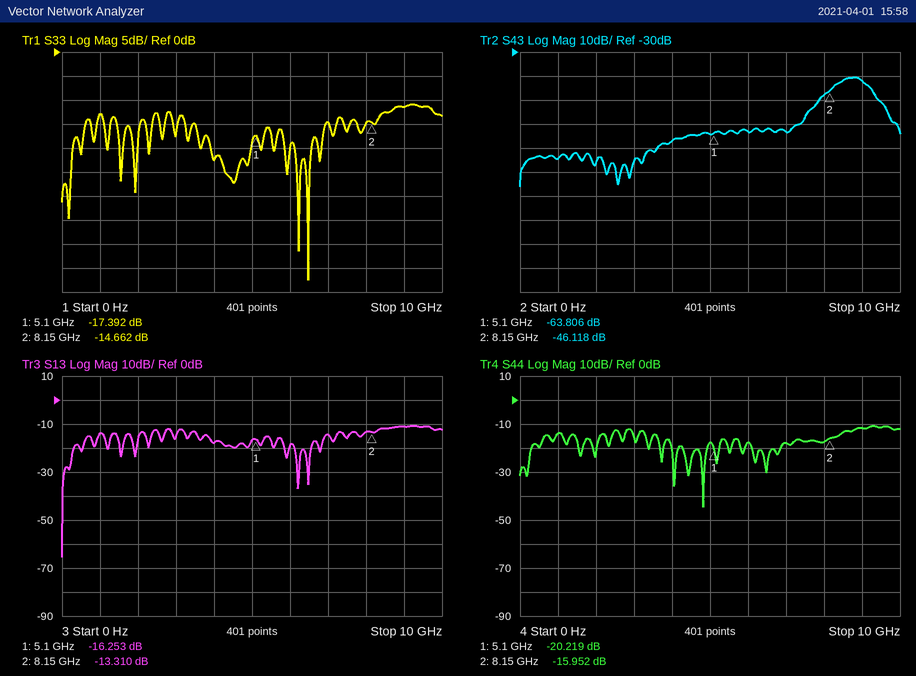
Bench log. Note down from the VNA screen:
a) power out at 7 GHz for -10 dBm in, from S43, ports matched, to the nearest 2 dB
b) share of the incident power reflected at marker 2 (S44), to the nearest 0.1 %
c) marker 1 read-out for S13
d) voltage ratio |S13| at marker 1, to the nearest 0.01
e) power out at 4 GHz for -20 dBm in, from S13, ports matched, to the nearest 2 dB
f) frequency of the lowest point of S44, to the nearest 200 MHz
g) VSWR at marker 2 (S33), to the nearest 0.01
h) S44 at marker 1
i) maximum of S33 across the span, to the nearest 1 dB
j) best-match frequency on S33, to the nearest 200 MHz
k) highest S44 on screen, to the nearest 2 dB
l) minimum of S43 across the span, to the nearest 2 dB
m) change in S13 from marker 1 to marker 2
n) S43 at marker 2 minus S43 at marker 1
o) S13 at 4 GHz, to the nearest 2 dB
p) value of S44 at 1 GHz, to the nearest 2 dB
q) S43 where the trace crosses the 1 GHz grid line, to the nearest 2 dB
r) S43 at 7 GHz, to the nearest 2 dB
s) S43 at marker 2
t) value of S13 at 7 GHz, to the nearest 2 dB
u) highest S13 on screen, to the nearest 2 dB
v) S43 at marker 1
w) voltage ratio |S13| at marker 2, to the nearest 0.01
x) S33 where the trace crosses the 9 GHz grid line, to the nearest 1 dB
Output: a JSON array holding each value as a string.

["-74 dBm", "2.5 %", "-16.253 dB", "0.15", "-38 dBm", "4.8 GHz", "1.45", "-20.219 dB", "-11 dB", "6.4 GHz", "-10 dB", "-86 dB", "2.943 dB", "17.688 dB", "-18 dB", "-14 dB", "-74 dB", "-64 dB", "-46.118 dB", "-14 dB", "-10 dB", "-63.806 dB", "0.22", "-11 dB"]
